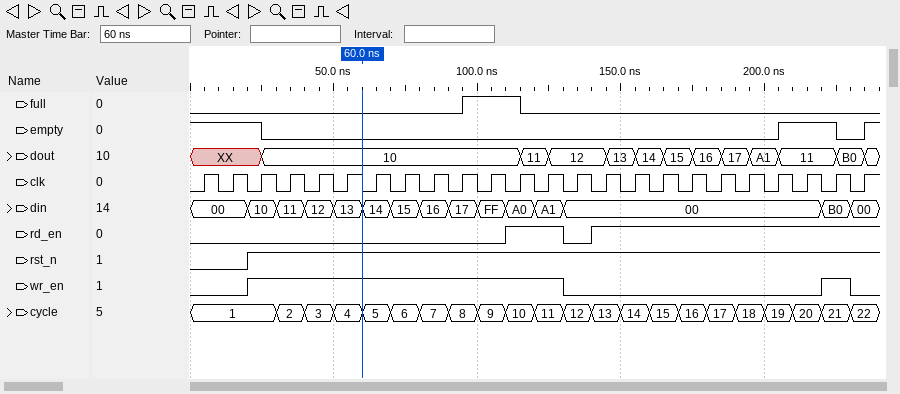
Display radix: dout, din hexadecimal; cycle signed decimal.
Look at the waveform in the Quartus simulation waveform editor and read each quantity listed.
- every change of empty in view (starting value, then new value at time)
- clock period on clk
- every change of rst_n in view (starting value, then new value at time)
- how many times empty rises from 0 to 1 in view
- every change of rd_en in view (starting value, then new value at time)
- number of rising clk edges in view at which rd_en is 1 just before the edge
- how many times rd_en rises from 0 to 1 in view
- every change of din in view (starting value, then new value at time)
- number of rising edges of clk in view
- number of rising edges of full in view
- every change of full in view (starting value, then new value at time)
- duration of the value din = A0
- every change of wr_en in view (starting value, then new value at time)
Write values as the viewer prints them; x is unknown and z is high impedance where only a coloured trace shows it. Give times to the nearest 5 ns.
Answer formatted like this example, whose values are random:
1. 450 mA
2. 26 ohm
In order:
1. 1, 0 at 25 ns, 1 at 205 ns, 0 at 225 ns, 1 at 235 ns
2. 10 ns
3. 0, 1 at 20 ns
4. 2
5. 0, 1 at 110 ns, 0 at 130 ns, 1 at 140 ns
6. 12
7. 2
8. 00, 10 at 20 ns, 11 at 30 ns, 12 at 40 ns, 13 at 50 ns, 14 at 60 ns, 15 at 70 ns, 16 at 80 ns, 17 at 90 ns, FF at 100 ns, A0 at 110 ns, A1 at 120 ns, 00 at 130 ns, B0 at 220 ns, 00 at 230 ns
9. 24
10. 1
11. 0, 1 at 95 ns, 0 at 115 ns
12. 10 ns
13. 0, 1 at 20 ns, 0 at 130 ns, 1 at 220 ns, 0 at 230 ns
